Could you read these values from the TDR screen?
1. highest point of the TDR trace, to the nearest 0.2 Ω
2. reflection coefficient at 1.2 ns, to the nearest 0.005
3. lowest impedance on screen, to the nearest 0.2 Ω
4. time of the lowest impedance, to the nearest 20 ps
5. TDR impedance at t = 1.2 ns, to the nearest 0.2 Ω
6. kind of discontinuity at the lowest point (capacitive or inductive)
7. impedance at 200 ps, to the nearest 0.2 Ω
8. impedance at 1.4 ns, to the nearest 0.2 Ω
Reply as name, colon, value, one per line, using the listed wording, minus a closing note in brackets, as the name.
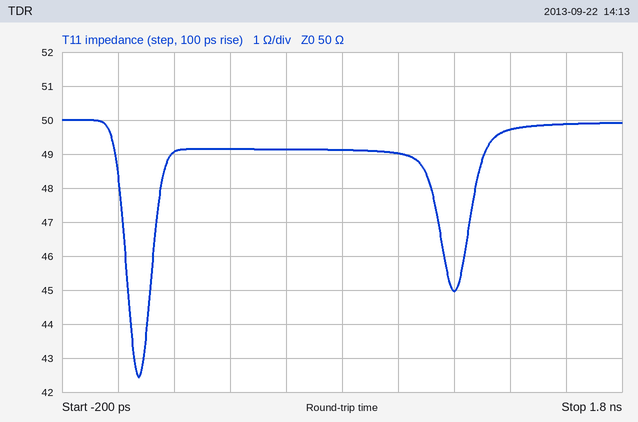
highest point of the TDR trace, to the nearest 0.2 Ω: 50.0 Ω
reflection coefficient at 1.2 ns, to the nearest 0.005: -0.055
lowest impedance on screen, to the nearest 0.2 Ω: 42.4 Ω
time of the lowest impedance, to the nearest 20 ps: 80 ps
TDR impedance at t = 1.2 ns, to the nearest 0.2 Ω: 45.0 Ω
kind of discontinuity at the lowest point: capacitive
impedance at 200 ps, to the nearest 0.2 Ω: 49.0 Ω
impedance at 1.4 ns, to the nearest 0.2 Ω: 49.8 Ω
